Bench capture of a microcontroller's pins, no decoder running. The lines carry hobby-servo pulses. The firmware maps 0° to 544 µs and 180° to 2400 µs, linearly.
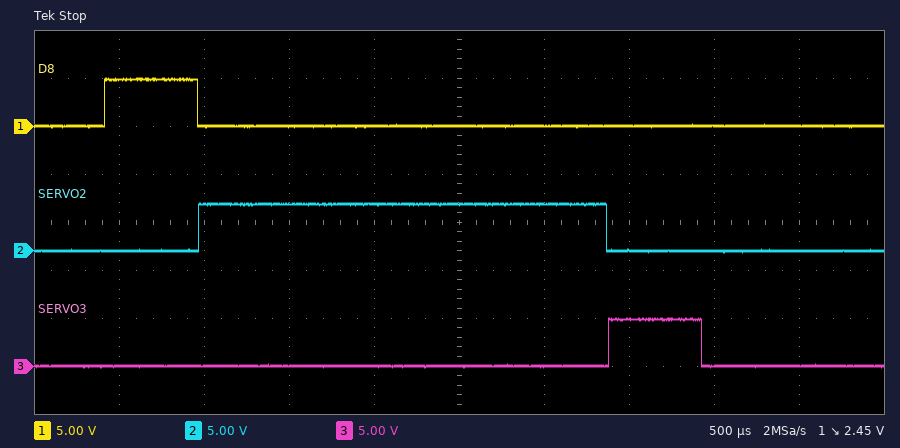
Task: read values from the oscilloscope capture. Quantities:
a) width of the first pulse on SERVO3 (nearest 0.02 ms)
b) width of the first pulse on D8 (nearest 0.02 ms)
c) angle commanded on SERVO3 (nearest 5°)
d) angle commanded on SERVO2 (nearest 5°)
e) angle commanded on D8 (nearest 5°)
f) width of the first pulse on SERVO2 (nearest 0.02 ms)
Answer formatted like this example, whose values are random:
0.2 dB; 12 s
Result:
0.54 ms; 0.54 ms; 0°; 180°; 0°; 2.40 ms
